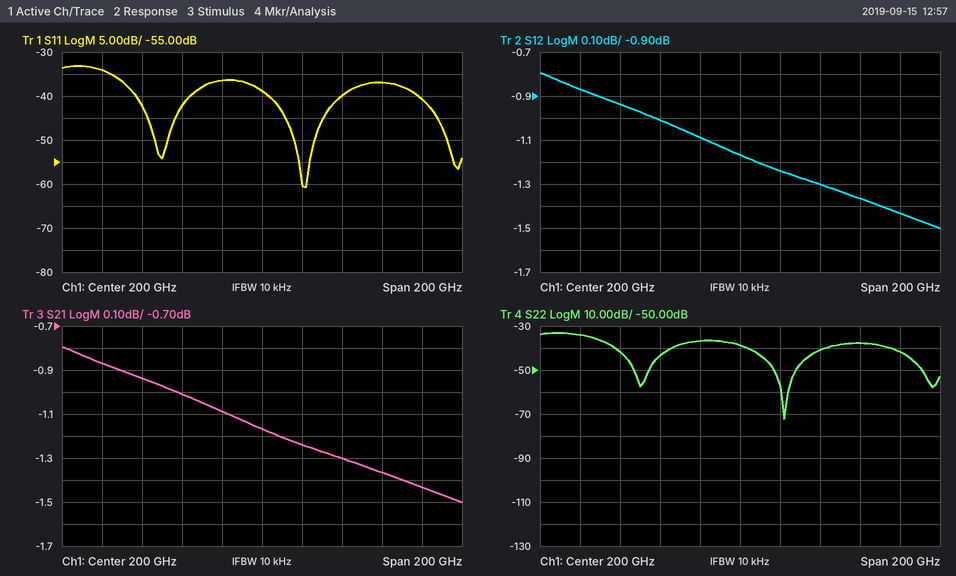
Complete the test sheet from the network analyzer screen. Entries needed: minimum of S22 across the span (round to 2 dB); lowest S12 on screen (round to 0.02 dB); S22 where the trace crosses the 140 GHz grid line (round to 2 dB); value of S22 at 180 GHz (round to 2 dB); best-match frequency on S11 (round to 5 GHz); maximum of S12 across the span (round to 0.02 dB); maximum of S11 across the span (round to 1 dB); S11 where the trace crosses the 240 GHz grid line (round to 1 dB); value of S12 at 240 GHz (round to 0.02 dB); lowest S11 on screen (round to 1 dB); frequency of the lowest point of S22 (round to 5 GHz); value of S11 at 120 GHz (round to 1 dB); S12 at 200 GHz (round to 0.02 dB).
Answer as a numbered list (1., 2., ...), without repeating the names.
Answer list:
1. -72 dB
2. -1.50 dB
3. -42 dB
4. -36 dB
5. 220 GHz
6. -0.80 dB
7. -33 dB
8. -40 dB
9. -1.30 dB
10. -61 dB
11. 220 GHz
12. -34 dB
13. -1.16 dB
